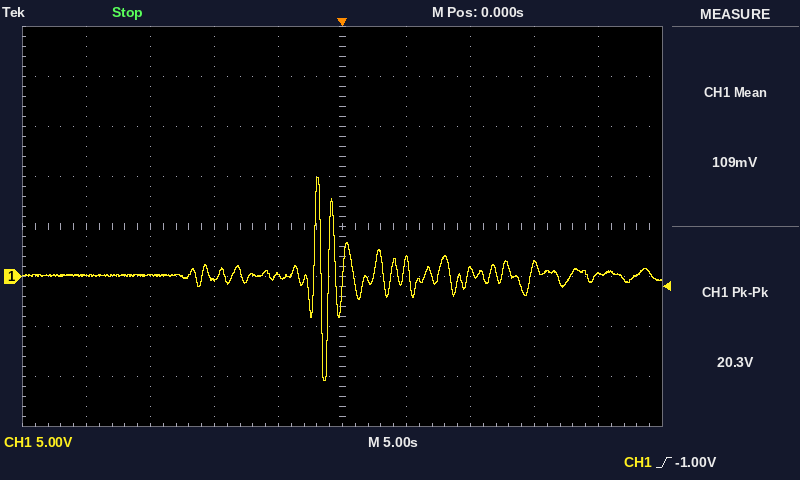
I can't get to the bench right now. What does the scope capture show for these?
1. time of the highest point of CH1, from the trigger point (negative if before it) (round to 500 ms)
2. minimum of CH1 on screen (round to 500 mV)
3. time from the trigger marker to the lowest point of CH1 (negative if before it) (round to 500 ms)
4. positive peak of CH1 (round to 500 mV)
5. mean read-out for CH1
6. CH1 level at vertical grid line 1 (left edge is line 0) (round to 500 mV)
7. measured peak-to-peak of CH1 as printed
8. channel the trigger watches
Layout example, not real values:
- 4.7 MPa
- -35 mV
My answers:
- -2.0 s
- -10.5 V
- -1.5 s
- 10.0 V
- 109 mV
- 0.0 V
- 20.3 V
- CH1
